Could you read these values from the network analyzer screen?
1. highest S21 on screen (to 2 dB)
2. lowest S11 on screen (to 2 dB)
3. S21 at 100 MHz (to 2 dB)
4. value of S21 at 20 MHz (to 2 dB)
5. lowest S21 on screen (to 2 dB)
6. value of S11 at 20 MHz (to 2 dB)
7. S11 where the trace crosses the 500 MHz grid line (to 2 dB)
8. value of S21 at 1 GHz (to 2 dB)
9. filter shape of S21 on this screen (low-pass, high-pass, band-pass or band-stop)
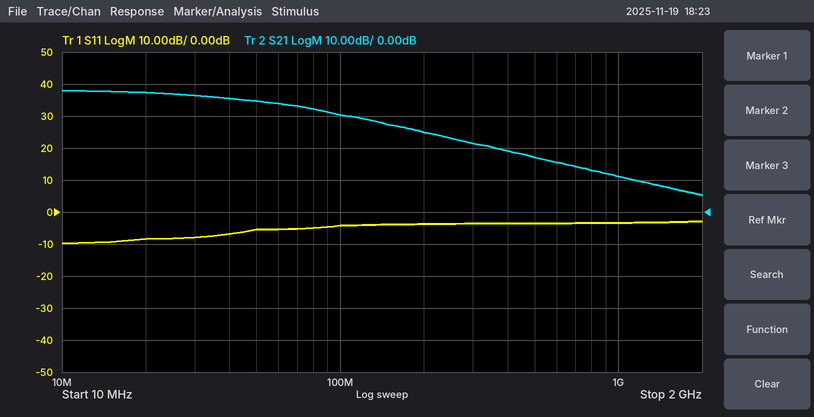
38 dB
-10 dB
30 dB
38 dB
6 dB
-8 dB
-4 dB
12 dB
low-pass
